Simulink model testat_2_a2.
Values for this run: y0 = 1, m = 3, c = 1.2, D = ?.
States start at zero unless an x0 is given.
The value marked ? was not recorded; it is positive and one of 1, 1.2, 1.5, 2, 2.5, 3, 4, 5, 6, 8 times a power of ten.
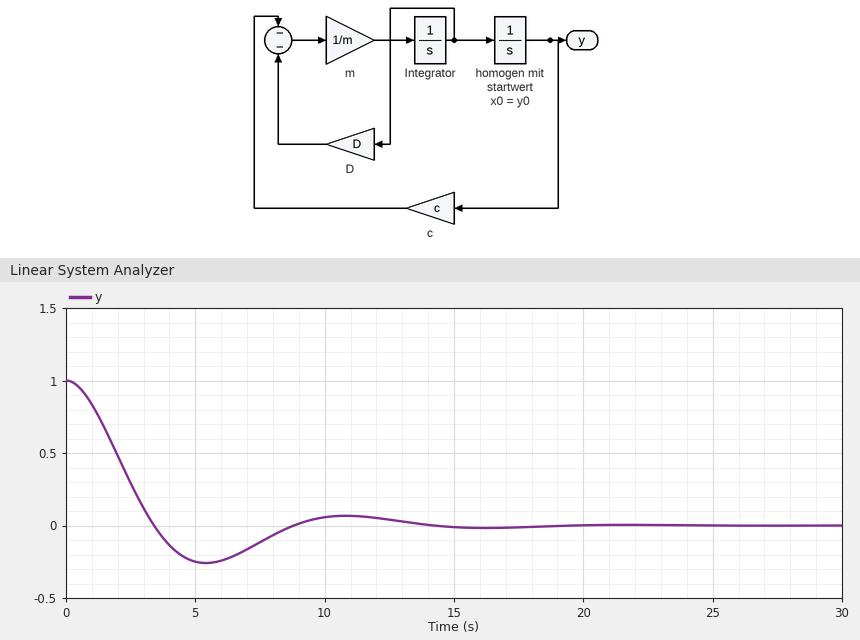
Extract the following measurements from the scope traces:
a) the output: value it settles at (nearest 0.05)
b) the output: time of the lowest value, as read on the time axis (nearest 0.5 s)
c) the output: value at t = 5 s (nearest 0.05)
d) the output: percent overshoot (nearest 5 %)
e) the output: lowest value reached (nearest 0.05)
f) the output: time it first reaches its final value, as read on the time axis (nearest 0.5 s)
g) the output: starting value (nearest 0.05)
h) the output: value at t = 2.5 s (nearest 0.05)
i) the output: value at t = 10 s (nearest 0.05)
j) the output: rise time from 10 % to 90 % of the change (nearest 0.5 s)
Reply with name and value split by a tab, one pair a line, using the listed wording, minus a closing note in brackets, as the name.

the output: value it settles at	0.00
the output: time of the lowest value, as read on the time axis	5.5 s
the output: value at t = 5 s	-0.25
the output: percent overshoot	25 %
the output: lowest value reached	-0.25
the output: time it first reaches its final value, as read on the time axis	3.5 s
the output: starting value	1.00
the output: value at t = 2.5 s	0.30
the output: value at t = 10 s	0.05
the output: rise time from 10 % to 90 % of the change	2.5 s
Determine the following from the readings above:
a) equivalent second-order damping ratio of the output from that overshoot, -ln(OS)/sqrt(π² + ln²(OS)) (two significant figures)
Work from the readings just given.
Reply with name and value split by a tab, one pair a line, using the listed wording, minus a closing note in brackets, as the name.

equivalent second-order damping ratio of the output from that overshoot, -ln(OS)/sqrt(π² + ln²(OS))	0.40
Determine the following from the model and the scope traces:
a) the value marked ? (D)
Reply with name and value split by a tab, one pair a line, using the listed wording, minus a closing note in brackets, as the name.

the value marked ?	1.5
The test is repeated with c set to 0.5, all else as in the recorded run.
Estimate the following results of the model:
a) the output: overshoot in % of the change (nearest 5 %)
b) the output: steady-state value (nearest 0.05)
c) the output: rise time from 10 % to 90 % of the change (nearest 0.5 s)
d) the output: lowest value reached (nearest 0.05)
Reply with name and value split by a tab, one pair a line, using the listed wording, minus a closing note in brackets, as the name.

the output: overshoot in % of the change	10 %
the output: steady-state value	0.00
the output: rise time from 10 % to 90 % of the change	4.5 s
the output: lowest value reached	-0.10
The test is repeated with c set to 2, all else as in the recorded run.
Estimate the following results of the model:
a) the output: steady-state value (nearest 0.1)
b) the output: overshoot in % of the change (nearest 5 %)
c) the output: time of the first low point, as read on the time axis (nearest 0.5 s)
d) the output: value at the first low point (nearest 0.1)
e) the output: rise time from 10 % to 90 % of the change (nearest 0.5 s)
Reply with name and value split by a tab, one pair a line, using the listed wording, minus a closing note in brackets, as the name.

the output: steady-state value	0.0
the output: overshoot in % of the change	35 %
the output: time of the first low point, as read on the time axis	4.0 s
the output: value at the first low point	-0.4
the output: rise time from 10 % to 90 % of the change	1.5 s
